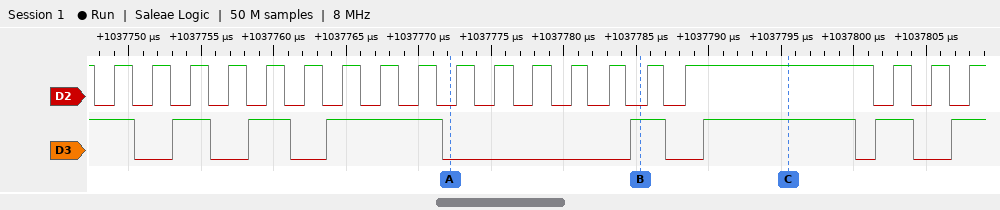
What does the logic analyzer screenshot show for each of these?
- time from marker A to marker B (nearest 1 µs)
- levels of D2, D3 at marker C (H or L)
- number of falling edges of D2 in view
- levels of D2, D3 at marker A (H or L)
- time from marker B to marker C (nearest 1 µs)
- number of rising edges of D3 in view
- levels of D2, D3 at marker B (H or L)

13 µs
D2=H, D3=H
19
D2=L, D3=L
10 µs
7
D2=L, D3=H
